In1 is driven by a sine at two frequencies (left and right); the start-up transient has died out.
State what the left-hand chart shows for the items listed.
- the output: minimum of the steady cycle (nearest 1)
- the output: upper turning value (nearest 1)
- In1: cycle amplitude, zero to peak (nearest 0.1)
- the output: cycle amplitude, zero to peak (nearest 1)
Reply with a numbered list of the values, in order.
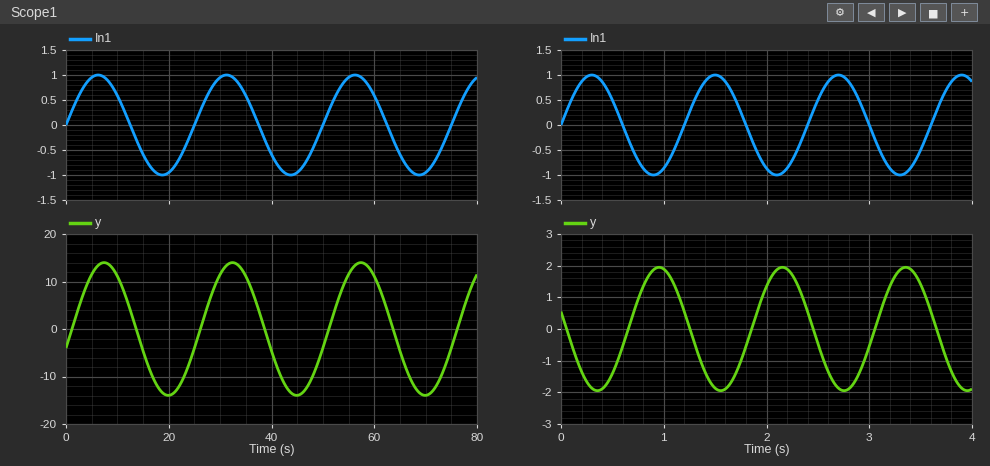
1. -14
2. 14
3. 1.0
4. 14
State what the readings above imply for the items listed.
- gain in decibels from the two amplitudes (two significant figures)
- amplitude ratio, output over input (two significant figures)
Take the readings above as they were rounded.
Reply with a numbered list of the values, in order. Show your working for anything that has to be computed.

1. 20 log10(14 / 1) = 23 dB
2. 14 / 1 = 14
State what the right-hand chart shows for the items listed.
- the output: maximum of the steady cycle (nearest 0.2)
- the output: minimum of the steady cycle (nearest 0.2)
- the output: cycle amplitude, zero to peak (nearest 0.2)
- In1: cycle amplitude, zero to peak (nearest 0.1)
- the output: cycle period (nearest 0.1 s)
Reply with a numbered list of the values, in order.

1. 2.0
2. -2.0
3. 2.0
4. 1.0
5. 1.2 s
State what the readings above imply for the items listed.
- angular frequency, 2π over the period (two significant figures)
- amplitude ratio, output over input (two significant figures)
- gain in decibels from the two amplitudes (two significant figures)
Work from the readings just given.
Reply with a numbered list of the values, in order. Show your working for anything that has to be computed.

1. 2π / 1.2 = 5.2 rad/s
2. 2 / 1 = 2.0
3. 20 log10(2 / 1) = 6.0 dB
